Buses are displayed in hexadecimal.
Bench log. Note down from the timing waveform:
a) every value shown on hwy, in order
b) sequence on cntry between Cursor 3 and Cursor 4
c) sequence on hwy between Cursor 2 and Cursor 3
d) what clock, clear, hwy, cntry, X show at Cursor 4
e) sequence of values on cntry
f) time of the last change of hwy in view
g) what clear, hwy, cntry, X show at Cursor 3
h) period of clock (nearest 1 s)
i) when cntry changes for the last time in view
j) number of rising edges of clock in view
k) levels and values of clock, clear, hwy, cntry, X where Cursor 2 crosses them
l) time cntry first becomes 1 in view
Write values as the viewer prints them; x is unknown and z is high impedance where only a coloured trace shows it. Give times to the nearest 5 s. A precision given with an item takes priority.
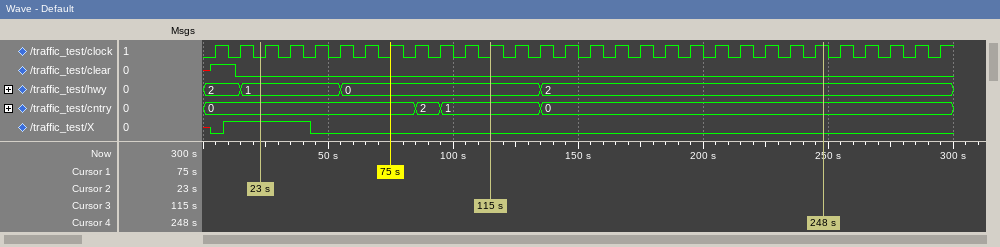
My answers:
2, 1, 0, 2
1, 0
1, 0
clock=1, clear=0, hwy=2, cntry=0, X=0
0, 2, 1, 0
135 s
clear=0, hwy=0, cntry=1, X=0
10 s
135 s
30
clock=0, clear=0, hwy=1, cntry=0, X=1
95 s
